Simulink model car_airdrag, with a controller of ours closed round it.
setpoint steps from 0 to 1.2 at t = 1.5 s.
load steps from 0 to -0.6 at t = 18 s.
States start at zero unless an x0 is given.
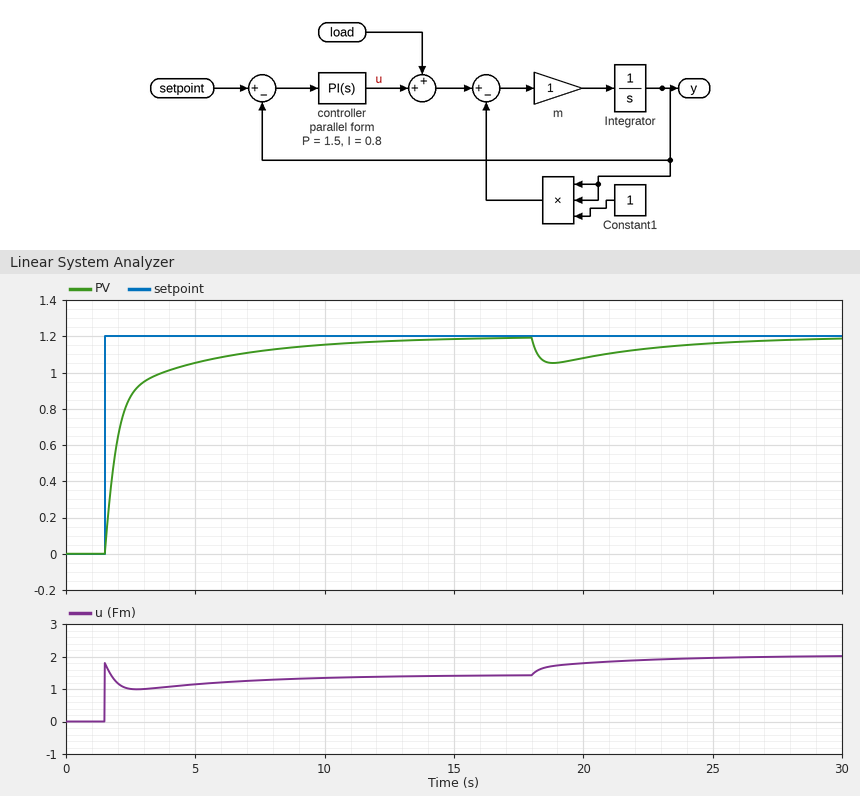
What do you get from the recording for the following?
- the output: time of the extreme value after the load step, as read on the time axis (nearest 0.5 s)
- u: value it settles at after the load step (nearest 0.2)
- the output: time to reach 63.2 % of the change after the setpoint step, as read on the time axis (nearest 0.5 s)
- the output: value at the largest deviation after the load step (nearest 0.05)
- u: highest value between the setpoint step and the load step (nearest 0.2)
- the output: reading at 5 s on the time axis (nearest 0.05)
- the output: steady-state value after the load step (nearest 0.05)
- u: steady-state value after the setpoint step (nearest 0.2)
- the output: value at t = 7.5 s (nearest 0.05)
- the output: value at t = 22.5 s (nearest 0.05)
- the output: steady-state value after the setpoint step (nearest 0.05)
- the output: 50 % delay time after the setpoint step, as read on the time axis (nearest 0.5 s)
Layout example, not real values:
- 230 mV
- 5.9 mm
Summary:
- 19.0 s
- 2.0
- 2.0 s
- 1.05
- 1.8
- 1.05
- 1.20
- 1.4
- 1.10
- 1.15
- 1.20
- 2.0 s
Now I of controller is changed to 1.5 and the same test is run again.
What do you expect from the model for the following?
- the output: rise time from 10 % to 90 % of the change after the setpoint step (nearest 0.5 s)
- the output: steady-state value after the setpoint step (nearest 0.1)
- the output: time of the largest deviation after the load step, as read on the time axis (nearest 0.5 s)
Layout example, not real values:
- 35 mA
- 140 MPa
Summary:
- 1.5 s
- 1.2
- 18.5 s
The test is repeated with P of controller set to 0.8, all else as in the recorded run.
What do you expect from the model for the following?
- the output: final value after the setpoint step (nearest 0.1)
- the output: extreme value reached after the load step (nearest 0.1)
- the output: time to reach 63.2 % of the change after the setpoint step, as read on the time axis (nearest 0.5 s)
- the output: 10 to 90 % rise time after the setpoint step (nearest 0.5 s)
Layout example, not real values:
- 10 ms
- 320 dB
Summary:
- 1.2
- 1.0
- 2.5 s
- 3.5 s
